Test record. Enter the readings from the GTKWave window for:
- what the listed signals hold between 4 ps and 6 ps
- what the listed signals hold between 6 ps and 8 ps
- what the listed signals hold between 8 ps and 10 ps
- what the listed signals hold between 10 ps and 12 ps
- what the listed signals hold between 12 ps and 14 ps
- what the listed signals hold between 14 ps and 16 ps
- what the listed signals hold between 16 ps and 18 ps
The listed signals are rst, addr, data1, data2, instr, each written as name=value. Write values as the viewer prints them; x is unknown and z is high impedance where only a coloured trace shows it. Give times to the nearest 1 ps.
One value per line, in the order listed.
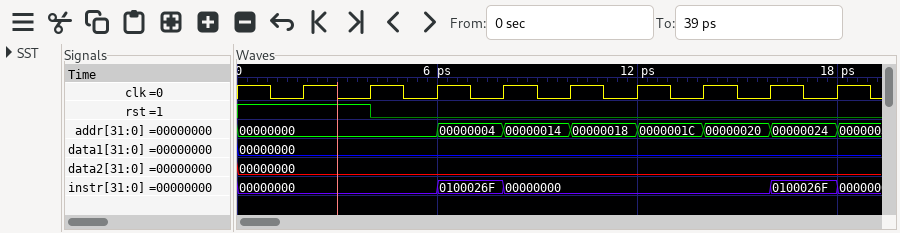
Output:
rst=0, addr=00000000, data1=00000000, data2=00000000, instr=00000000
rst=0, addr=00000004, data1=00000000, data2=00000000, instr=0100026F
rst=0, addr=00000014, data1=00000000, data2=00000000, instr=00000000
rst=0, addr=00000018, data1=00000000, data2=00000000, instr=00000000
rst=0, addr=0000001C, data1=00000000, data2=00000000, instr=00000000
rst=0, addr=00000020, data1=00000000, data2=00000000, instr=00000000
rst=0, addr=00000024, data1=00000000, data2=00000000, instr=0100026F
